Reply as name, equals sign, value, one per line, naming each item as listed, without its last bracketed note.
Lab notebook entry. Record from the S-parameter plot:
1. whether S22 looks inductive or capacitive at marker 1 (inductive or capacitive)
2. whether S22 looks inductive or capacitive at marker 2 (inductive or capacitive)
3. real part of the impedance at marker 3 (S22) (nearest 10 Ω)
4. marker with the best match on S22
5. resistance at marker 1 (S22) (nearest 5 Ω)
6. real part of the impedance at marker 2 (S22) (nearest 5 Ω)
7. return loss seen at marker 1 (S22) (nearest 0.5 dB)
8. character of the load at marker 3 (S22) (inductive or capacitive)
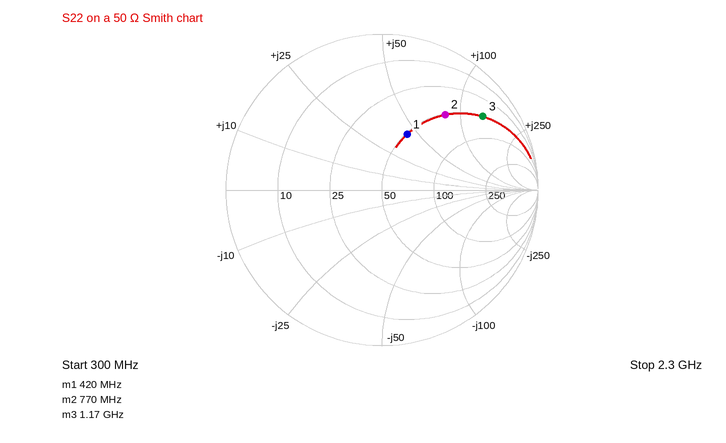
whether S22 looks inductive or capacitive at marker 1 = inductive
whether S22 looks inductive or capacitive at marker 2 = inductive
real part of the impedance at marker 3 (S22) = 50 Ω
marker with the best match on S22 = marker 1
resistance at marker 1 (S22) = 50 Ω
real part of the impedance at marker 2 (S22) = 50 Ω
return loss seen at marker 1 (S22) = 8.0 dB
character of the load at marker 3 (S22) = inductive
